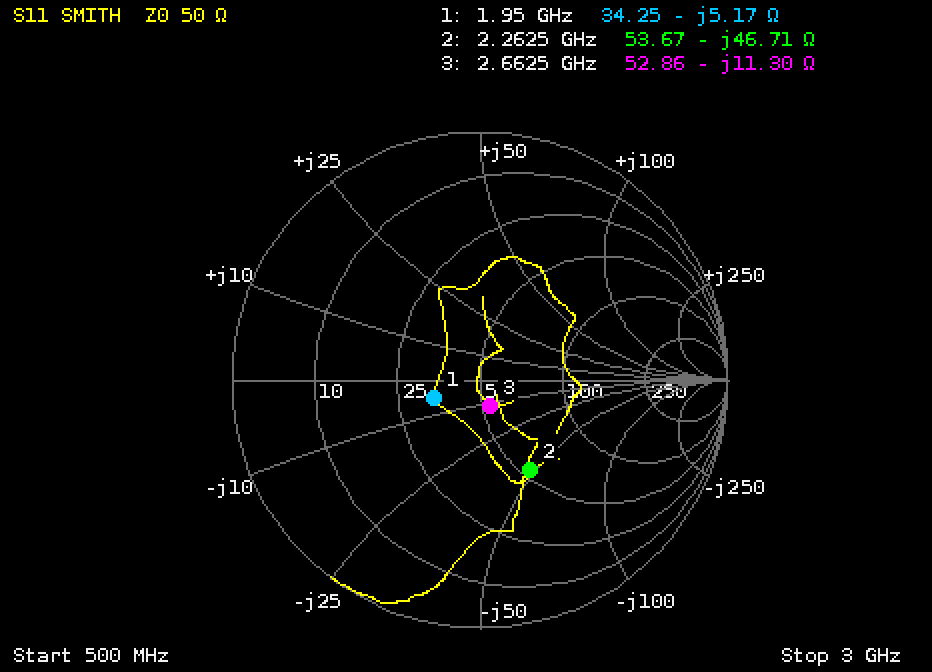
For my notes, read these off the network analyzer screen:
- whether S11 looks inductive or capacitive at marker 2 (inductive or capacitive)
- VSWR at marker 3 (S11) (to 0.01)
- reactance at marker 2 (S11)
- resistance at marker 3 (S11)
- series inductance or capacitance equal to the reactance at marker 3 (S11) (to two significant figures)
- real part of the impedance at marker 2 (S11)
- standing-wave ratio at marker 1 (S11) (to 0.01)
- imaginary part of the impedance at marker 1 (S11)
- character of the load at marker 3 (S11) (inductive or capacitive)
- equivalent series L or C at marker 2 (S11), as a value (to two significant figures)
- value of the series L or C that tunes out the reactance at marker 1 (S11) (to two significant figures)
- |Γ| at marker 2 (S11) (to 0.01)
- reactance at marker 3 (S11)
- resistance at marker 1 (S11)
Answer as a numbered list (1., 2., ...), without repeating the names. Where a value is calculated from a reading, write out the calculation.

1. capacitive
2. 1.25
3. -46.71 Ω
4. 52.86 Ω
5. C = 1/(2π × 2.6625 GHz × 11.3 Ω) ≈ 5.3 pF
6. 53.67 Ω
7. 1.49
8. -5.17 Ω
9. capacitive
10. C = 1/(2π × 2.2625 GHz × 46.71 Ω) ≈ 1.5 pF
11. L = 5.17 Ω/(2π × 1.95 GHz) ≈ 422 pH, so 420 pH to two significant figures
12. 0.41
13. -11.30 Ω
14. 34.25 Ω
